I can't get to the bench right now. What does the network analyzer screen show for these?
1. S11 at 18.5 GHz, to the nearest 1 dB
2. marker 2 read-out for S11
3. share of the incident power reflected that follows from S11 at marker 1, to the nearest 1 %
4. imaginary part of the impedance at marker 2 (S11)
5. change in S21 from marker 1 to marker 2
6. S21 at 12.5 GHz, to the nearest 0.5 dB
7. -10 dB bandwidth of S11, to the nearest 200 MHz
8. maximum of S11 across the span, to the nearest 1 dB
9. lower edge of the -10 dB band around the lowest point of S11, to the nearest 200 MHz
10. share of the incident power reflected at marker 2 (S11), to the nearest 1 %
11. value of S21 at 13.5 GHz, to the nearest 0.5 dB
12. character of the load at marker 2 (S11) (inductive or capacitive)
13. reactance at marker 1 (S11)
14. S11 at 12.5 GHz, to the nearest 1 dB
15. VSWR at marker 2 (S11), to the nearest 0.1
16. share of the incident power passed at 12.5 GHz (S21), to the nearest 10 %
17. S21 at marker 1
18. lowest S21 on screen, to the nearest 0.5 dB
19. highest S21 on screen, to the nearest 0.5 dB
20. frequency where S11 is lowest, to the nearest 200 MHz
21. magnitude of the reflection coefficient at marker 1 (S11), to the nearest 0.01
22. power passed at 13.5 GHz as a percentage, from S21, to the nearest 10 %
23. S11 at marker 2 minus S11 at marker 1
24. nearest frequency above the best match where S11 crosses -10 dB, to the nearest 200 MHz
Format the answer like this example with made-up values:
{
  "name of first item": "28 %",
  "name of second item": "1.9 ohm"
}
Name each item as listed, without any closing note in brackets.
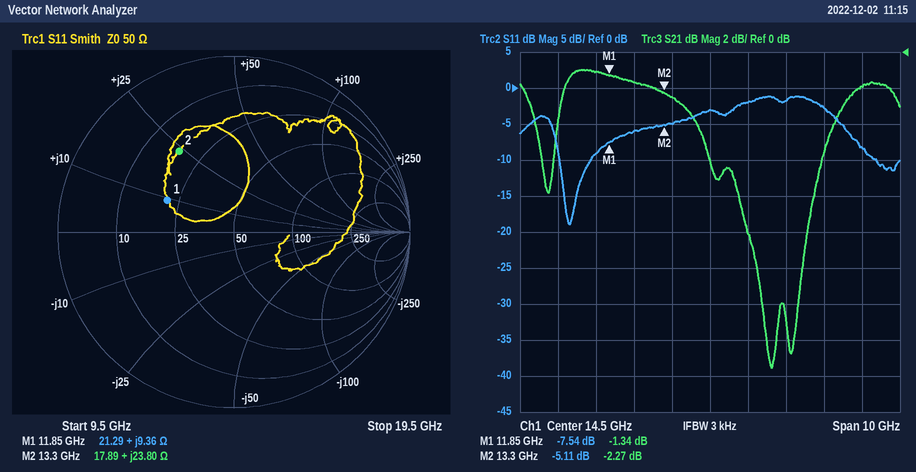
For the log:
{
  "S11 at 18.5 GHz, to the nearest 1 dB": "-8 dB",
  "marker 2 read-out for S11": "-5.11 dB",
  "share of the incident power reflected that follows from S11 at marker 1, to the nearest 1 %": "18 %",
  "imaginary part of the impedance at marker 2": "+23.80 Ω",
  "change in S21 from marker 1 to marker 2": "-0.93 dB",
  "S21 at 12.5 GHz, to the nearest 0.5 dB": "-1.5 dB",
  "-10 dB bandwidth of S11, to the nearest 200 MHz": "800 MHz",
  "maximum of S11 across the span, to the nearest 1 dB": "-1 dB",
  "lower edge of the -10 dB band around the lowest point of S11, to the nearest 200 MHz": "10.6 GHz",
  "share of the incident power reflected at marker 2 (S11), to the nearest 1 %": "31 %",
  "value of S21 at 13.5 GHz, to the nearest 0.5 dB": "-2.5 dB",
  "character of the load at marker 2 (S11)": "inductive",
  "reactance at marker 1": "+9.36 Ω",
  "S11 at 12.5 GHz, to the nearest 1 dB": "-6 dB",
  "VSWR at marker 2 (S11), to the nearest 0.1": "3.5",
  "share of the incident power passed at 12.5 GHz (S21), to the nearest 10 %": "70 %",
  "S21 at marker 1": "-1.34 dB",
  "lowest S21 on screen, to the nearest 0.5 dB": "-17.5 dB",
  "highest S21 on screen, to the nearest 0.5 dB": "-1.0 dB",
  "frequency where S11 is lowest, to the nearest 200 MHz": "10.8 GHz",
  "magnitude of the reflection coefficient at marker 1 (S11), to the nearest 0.01": "0.42",
  "power passed at 13.5 GHz as a percentage, from S21, to the nearest 10 %": "60 %",
  "S11 at marker 2 minus S11 at marker 1": "2.43 dB",
  "nearest frequency above the best match where S11 crosses -10 dB, to the nearest 200 MHz": "11.4 GHz"
}
